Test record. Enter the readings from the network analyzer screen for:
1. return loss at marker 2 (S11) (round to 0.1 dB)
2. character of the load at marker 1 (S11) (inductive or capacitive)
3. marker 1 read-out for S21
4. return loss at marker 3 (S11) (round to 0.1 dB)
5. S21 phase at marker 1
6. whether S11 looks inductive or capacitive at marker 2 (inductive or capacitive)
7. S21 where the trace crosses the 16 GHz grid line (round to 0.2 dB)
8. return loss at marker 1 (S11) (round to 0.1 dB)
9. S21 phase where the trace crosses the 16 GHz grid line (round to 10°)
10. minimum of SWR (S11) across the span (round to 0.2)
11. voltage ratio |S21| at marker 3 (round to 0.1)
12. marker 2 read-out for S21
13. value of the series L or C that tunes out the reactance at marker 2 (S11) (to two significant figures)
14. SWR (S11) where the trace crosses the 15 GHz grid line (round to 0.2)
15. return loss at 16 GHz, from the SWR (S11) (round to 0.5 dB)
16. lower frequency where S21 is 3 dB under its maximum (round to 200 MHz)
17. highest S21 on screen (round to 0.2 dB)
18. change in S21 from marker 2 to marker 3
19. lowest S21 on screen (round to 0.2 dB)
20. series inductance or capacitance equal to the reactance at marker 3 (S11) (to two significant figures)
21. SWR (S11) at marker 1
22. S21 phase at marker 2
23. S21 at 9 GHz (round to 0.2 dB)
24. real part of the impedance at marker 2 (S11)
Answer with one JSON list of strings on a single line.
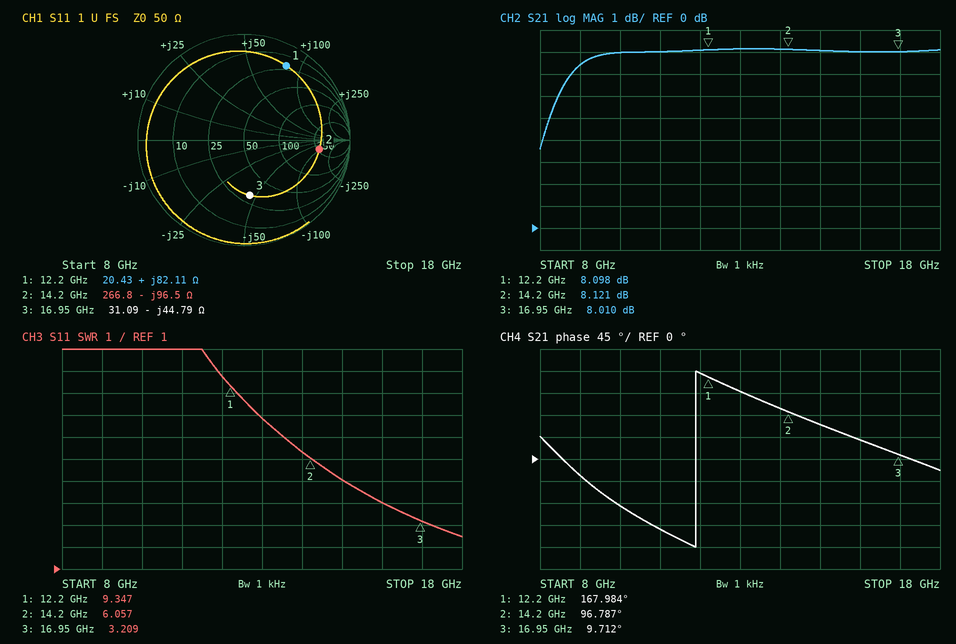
["2.9 dB", "inductive", "8.098 dB", "5.6 dB", "167.984°", "capacitive", "8.0 dB", "1.9 dB", "40°", "2.4", "2.5", "8.121 dB", "1.1 nH", "5.0", "4.5 dB", "8.2 GHz", "8.2 dB", "-0.111 dB", "3.6 dB", "210 fF", "9.347", "96.787°", "7.4 dB", "266.8 Ω"]
